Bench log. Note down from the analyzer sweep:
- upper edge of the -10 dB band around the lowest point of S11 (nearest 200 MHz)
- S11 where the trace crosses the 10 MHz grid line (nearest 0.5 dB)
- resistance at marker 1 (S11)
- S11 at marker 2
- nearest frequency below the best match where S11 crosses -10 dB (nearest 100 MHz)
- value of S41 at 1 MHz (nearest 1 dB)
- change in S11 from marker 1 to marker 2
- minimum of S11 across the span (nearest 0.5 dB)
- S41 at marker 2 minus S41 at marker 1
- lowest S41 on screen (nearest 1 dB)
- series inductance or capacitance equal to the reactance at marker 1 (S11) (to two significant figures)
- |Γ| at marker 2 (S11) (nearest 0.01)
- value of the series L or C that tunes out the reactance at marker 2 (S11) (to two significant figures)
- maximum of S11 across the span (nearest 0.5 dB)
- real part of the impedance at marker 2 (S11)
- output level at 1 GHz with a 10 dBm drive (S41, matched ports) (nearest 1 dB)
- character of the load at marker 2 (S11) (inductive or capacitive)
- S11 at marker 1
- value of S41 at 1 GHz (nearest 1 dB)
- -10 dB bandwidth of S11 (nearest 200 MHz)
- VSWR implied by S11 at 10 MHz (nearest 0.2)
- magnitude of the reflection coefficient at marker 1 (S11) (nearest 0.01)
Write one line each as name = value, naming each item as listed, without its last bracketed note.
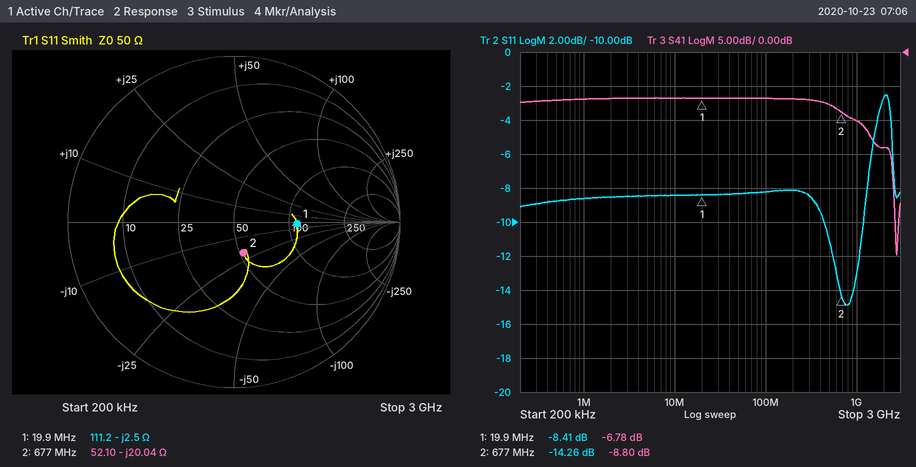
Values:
upper edge of the -10 dB band around the lowest point of S11 = 1.2 GHz
S11 where the trace crosses the 10 MHz grid line = -8.5 dB
resistance at marker 1 = 111.2 Ω
S11 at marker 2 = -14.26 dB
nearest frequency below the best match where S11 crosses -10 dB = 400 MHz
value of S41 at 1 MHz = -7 dB
change in S11 from marker 1 to marker 2 = -5.85 dB
minimum of S11 across the span = -15.0 dB
S41 at marker 2 minus S41 at marker 1 = -2.02 dB
lowest S41 on screen = -30 dB
series inductance or capacitance equal to the reactance at marker 1 (S11) = 3.2 nF
|Γ| at marker 2 (S11) = 0.19
value of the series L or C that tunes out the reactance at marker 2 (S11) = 4.7 nH
maximum of S11 across the span = -2.5 dB
real part of the impedance at marker 2 = 52.10 Ω
output level at 1 GHz with a 10 dBm drive (S41, matched ports) = 0 dBm
character of the load at marker 2 (S11) = capacitive
S11 at marker 1 = -8.41 dB
value of S41 at 1 GHz = -10 dB
-10 dB bandwidth of S11 = 800 MHz
VSWR implied by S11 at 10 MHz = 2.2
magnitude of the reflection coefficient at marker 1 (S11) = 0.38
